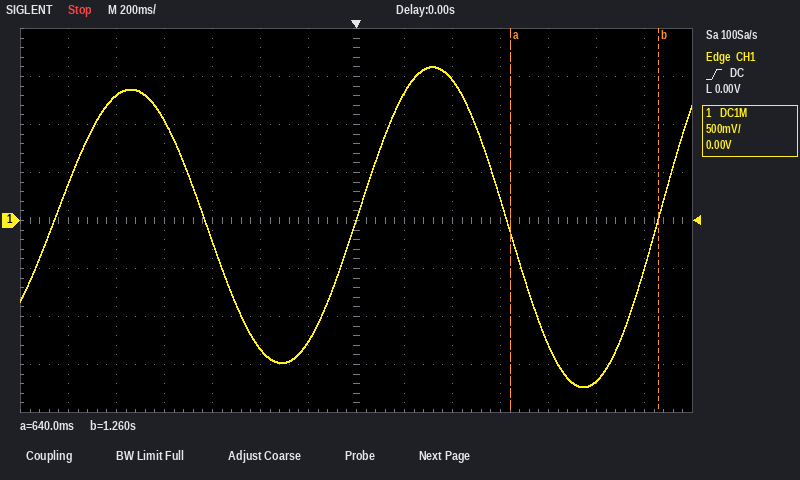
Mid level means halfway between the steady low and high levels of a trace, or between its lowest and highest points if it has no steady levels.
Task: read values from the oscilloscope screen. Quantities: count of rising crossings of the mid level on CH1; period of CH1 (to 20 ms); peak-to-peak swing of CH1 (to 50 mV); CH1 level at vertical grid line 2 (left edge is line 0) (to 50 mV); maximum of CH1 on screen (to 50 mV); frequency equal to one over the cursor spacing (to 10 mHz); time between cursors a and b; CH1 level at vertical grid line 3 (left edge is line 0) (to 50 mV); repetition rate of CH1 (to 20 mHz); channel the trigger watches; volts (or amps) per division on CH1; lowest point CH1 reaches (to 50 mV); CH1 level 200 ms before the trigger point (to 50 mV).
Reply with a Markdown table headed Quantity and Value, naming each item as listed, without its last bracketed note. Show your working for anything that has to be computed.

| Quantity | Value |
|---|---|
| count of rising crossings of the mid level on CH1 | 3 |
| period of CH1 | 1.26 s |
| peak-to-peak swing of CH1 | 1.60 V − (-1.75 V) = 3.35 V |
| CH1 level at vertical grid line 2 (left edge is line 0) | 1.30 V |
| maximum of CH1 on screen | 1.60 V |
| frequency equal to one over the cursor spacing | 1 / 620 ms ≈ 1.61 Hz |
| time between cursors a and b | 1.26 s − (640 ms) = 620 ms |
| CH1 level at vertical grid line 3 (left edge is line 0) | 1.05 V |
| repetition rate of CH1 | 1 / 1.26 s ≈ 794 mHz, so 800 mHz to the nearest 20 mHz |
| channel the trigger watches | CH1 |
| volts (or amps) per division on CH1 | 500 mV |
| lowest point CH1 reaches | -1.75 V |
| CH1 level 200 ms before the trigger point | -1.25 V |
